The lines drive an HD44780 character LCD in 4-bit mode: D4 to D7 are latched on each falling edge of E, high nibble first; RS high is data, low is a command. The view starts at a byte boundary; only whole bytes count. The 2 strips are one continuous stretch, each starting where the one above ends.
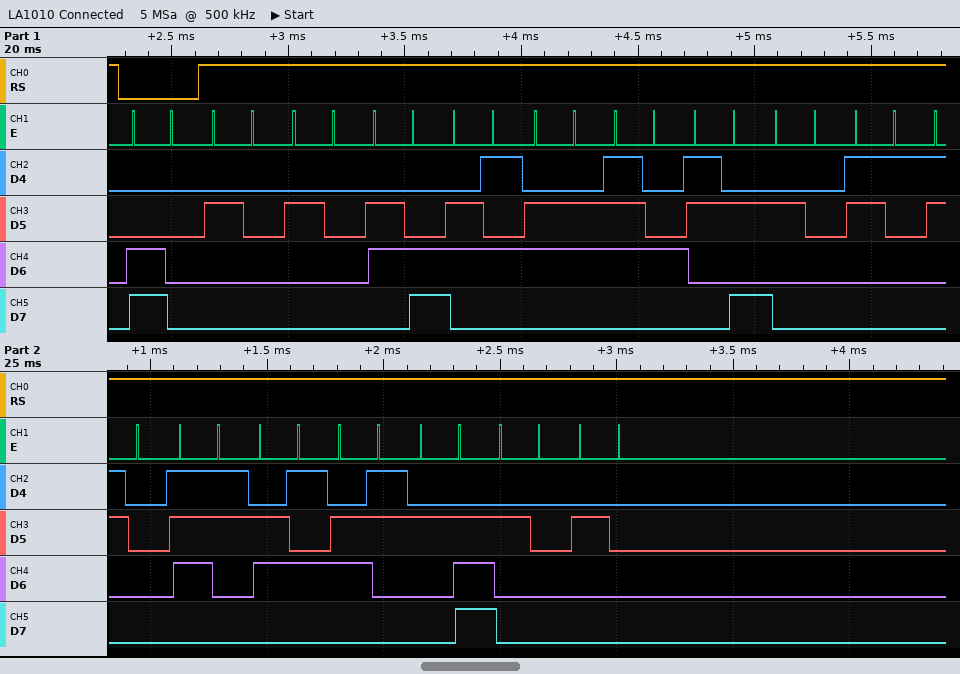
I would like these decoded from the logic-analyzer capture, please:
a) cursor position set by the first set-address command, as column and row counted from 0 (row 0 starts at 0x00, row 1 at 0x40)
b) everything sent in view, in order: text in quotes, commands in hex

column 0, row 1
0xC0 "  left: 10sec.  "
